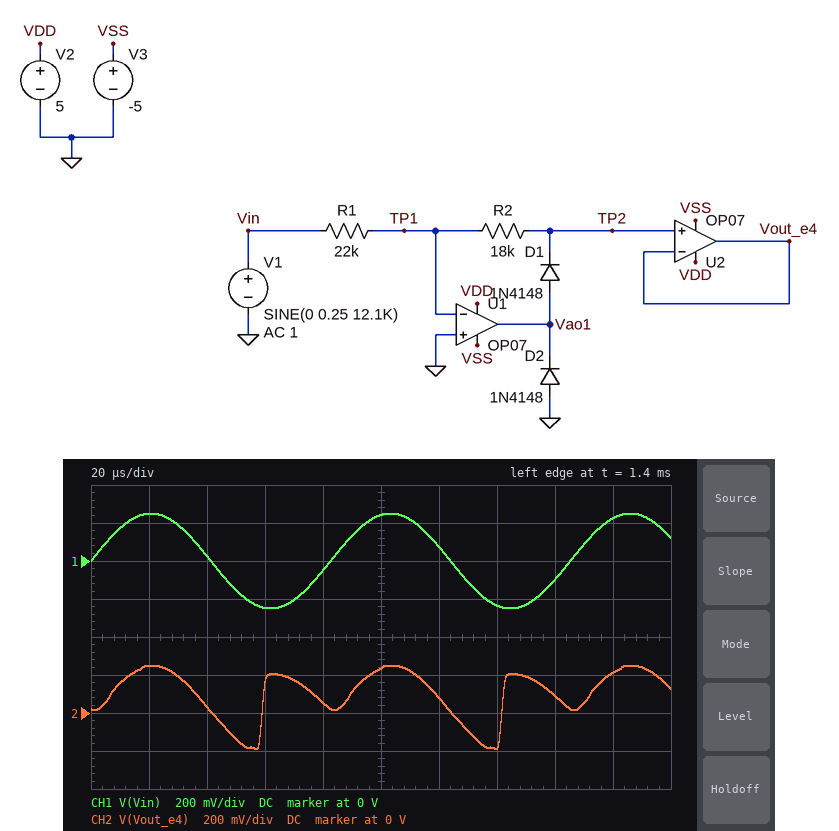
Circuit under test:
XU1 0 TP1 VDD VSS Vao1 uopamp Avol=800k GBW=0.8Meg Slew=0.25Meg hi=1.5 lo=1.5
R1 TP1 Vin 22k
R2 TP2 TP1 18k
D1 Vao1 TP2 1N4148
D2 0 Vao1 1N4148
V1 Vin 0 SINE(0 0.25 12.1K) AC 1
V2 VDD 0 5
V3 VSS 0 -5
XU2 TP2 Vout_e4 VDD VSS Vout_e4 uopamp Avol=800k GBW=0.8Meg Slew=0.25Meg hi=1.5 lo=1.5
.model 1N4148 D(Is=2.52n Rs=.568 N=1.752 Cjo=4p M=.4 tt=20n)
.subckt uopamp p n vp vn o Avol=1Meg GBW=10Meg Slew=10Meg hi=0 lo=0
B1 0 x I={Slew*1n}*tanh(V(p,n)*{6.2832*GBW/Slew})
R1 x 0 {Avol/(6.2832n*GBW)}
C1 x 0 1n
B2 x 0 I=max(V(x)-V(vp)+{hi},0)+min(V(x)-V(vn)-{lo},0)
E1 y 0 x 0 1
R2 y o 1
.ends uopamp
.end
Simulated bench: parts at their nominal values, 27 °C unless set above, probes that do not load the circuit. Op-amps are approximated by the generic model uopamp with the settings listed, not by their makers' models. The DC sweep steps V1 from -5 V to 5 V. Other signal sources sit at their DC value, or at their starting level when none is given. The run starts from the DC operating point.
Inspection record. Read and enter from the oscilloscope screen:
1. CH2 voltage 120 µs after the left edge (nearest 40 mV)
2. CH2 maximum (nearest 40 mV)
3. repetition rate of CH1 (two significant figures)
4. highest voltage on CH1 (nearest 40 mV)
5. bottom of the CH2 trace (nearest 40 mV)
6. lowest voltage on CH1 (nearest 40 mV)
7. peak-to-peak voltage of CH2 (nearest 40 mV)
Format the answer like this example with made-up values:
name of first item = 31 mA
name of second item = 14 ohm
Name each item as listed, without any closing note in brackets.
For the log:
CH2 voltage 120 µs after the left edge = 80 mV
CH2 maximum = 240 mV
repetition rate of CH1 = 12 kHz
highest voltage on CH1 = 240 mV
bottom of the CH2 trace = -200 mV
lowest voltage on CH1 = -240 mV
peak-to-peak voltage of CH2 = 440 mV
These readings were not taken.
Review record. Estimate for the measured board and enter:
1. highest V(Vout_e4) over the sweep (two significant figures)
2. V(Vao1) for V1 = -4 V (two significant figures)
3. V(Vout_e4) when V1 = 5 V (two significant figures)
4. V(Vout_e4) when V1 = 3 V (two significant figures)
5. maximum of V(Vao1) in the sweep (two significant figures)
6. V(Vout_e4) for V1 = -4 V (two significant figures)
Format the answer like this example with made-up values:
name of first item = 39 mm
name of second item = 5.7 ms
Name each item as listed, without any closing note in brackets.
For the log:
highest V(Vout_e4) over the sweep = 3.5 V
V(Vao1) for V1 = -4 V = 3.5 V
V(Vout_e4) when V1 = 5 V = 3.5 V
V(Vout_e4) when V1 = 3 V = 3.0 V
maximum of V(Vao1) in the sweep = 3.5 V
V(Vout_e4) for V1 = -4 V = 3.0 V
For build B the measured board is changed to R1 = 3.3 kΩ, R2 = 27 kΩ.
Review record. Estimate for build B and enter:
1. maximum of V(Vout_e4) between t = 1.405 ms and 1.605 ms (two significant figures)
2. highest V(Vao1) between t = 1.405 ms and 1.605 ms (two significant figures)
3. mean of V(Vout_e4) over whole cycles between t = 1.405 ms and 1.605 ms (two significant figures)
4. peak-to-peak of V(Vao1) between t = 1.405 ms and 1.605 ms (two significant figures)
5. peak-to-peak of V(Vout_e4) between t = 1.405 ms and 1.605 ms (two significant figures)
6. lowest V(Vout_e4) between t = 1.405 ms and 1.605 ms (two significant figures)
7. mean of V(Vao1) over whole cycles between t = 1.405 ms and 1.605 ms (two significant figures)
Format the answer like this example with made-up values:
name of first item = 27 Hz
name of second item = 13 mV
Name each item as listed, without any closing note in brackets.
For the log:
maximum of V(Vout_e4) between t = 1.405 ms and 1.605 ms = 1.8 V
highest V(Vao1) between t = 1.405 ms and 1.605 ms = 2.3 V
mean of V(Vout_e4) over whole cycles between t = 1.405 ms and 1.605 ms = 390 mV
peak-to-peak of V(Vao1) between t = 1.405 ms and 1.605 ms = 4.1 V
peak-to-peak of V(Vout_e4) between t = 1.405 ms and 1.605 ms = 2.0 V
lowest V(Vout_e4) between t = 1.405 ms and 1.605 ms = -200 mV
mean of V(Vao1) over whole cycles between t = 1.405 ms and 1.605 ms = -460 mV
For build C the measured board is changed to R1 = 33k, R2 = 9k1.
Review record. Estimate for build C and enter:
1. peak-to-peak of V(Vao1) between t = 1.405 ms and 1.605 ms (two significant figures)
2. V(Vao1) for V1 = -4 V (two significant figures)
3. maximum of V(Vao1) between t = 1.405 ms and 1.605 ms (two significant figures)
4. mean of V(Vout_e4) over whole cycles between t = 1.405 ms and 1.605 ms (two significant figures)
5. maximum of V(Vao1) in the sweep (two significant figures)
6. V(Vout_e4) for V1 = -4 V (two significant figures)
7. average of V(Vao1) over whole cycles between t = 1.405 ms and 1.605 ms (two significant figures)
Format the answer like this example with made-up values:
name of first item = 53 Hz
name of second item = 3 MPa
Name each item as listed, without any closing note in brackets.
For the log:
peak-to-peak of V(Vao1) between t = 1.405 ms and 1.605 ms = 2.3 V
V(Vao1) for V1 = -4 V = 1.6 V
maximum of V(Vao1) between t = 1.405 ms and 1.605 ms = 430 mV
mean of V(Vout_e4) over whole cycles between t = 1.405 ms and 1.605 ms = 65 mV
maximum of V(Vao1) in the sweep = 1.9 V
V(Vout_e4) for V1 = -4 V = 1.1 V
average of V(Vao1) over whole cycles between t = 1.405 ms and 1.605 ms = -840 mV
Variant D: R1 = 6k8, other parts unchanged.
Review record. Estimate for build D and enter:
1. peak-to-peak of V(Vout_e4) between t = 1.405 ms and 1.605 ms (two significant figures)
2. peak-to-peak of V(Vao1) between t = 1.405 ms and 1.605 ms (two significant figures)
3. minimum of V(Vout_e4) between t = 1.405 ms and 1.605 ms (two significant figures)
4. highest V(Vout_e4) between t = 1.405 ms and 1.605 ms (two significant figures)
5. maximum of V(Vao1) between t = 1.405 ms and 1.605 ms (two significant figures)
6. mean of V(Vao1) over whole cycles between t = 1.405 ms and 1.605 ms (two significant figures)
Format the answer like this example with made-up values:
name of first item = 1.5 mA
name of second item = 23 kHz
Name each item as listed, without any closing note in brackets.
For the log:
peak-to-peak of V(Vout_e4) between t = 1.405 ms and 1.605 ms = 860 mV
peak-to-peak of V(Vao1) between t = 1.405 ms and 1.605 ms = 2.9 V
minimum of V(Vout_e4) between t = 1.405 ms and 1.605 ms = -200 mV
highest V(Vout_e4) between t = 1.405 ms and 1.605 ms = 650 mV
maximum of V(Vao1) between t = 1.405 ms and 1.605 ms = 1.1 V
mean of V(Vao1) over whole cycles between t = 1.405 ms and 1.605 ms = -710 mV
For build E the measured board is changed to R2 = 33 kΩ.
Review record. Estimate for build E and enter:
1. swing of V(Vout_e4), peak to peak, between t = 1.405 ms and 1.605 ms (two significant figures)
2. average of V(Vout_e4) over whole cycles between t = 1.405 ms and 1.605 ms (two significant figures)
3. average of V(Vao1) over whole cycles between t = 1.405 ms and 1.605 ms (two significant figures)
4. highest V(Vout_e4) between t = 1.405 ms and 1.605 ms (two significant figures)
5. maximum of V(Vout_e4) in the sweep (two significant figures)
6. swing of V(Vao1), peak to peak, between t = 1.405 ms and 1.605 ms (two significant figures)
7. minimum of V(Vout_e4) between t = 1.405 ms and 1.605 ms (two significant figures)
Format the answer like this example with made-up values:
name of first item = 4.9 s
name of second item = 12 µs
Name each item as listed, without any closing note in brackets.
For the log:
swing of V(Vout_e4), peak to peak, between t = 1.405 ms and 1.605 ms = 550 mV
average of V(Vout_e4) over whole cycles between t = 1.405 ms and 1.605 ms = 120 mV
average of V(Vao1) over whole cycles between t = 1.405 ms and 1.605 ms = -780 mV
highest V(Vout_e4) between t = 1.405 ms and 1.605 ms = 370 mV
maximum of V(Vout_e4) in the sweep = 3.5 V
swing of V(Vao1), peak to peak, between t = 1.405 ms and 1.605 ms = 2.6 V
minimum of V(Vout_e4) between t = 1.405 ms and 1.605 ms = -180 mV
